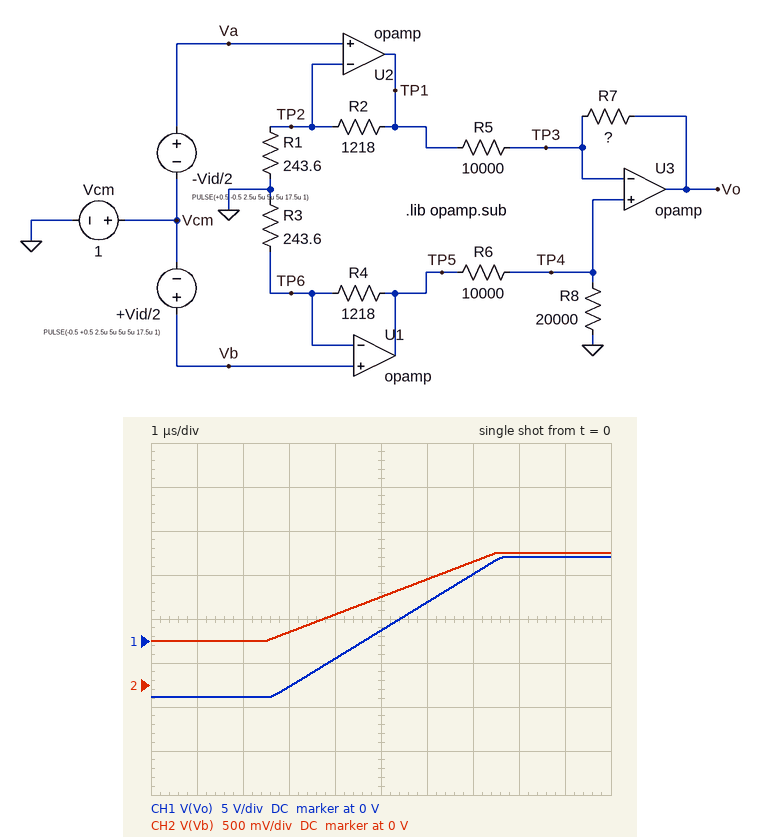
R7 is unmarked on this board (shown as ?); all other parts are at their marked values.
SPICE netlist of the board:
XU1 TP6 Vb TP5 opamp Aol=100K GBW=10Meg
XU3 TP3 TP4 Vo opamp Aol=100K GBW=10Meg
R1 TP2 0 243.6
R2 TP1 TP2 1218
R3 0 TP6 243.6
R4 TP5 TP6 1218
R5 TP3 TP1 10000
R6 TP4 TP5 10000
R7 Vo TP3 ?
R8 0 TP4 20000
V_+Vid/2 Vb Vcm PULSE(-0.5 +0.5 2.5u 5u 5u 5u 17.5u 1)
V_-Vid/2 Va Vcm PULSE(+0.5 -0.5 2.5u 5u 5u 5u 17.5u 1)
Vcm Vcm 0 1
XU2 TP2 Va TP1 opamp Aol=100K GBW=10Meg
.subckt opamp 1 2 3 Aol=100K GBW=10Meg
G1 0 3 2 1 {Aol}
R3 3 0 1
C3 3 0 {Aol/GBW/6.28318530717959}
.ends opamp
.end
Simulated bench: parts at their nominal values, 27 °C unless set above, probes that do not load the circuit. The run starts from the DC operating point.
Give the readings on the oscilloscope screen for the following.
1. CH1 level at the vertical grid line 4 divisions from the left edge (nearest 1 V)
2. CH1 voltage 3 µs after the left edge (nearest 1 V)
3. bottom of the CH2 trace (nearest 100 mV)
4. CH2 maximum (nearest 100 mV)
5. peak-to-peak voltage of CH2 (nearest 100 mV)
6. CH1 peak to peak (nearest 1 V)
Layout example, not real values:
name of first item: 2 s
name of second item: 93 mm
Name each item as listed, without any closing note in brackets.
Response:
CH1 level at the vertical grid line 4 divisions from the left edge: -2 V
CH1 voltage 3 µs after the left edge: -5 V
bottom of the CH2 trace: 500 mV
CH2 maximum: 1.5 V
peak-to-peak voltage of CH2: 1.0 V
CH1 peak to peak: 16 V
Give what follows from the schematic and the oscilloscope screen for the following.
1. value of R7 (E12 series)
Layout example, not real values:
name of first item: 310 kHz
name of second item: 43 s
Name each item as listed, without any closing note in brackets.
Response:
value of R7: 12 kΩ
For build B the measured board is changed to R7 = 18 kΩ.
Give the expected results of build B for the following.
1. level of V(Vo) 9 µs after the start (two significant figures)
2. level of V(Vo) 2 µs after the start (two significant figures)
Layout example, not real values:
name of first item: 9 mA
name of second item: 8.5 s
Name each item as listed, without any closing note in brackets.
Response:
level of V(Vo) 9 µs after the start: 11 V
level of V(Vo) 2 µs after the start: -11 V
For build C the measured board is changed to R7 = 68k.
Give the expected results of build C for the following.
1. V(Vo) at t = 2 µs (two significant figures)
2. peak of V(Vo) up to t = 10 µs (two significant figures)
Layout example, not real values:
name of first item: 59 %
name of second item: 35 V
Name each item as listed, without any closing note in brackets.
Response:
V(Vo) at t = 2 µs: -46 V
peak of V(Vo) up to t = 10 µs: 26 V
